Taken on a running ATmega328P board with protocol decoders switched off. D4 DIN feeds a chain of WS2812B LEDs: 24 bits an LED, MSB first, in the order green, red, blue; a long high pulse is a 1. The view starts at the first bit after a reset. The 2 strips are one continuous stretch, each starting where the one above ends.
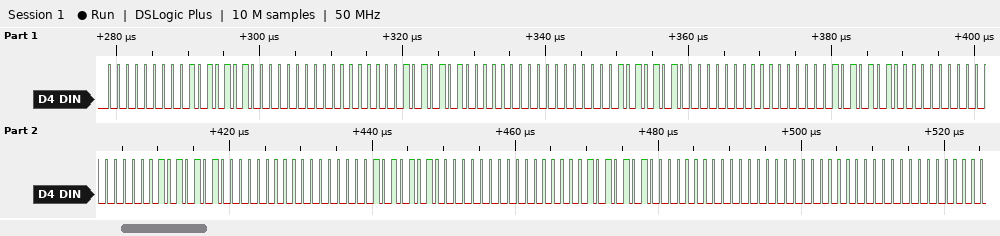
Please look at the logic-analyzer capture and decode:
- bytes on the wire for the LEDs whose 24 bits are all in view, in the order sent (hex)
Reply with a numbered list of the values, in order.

1. 00 55 00 00 55 00 00 55 00 00 55 00 00 55 00 00 55 00 00 55 00 00 00 00
